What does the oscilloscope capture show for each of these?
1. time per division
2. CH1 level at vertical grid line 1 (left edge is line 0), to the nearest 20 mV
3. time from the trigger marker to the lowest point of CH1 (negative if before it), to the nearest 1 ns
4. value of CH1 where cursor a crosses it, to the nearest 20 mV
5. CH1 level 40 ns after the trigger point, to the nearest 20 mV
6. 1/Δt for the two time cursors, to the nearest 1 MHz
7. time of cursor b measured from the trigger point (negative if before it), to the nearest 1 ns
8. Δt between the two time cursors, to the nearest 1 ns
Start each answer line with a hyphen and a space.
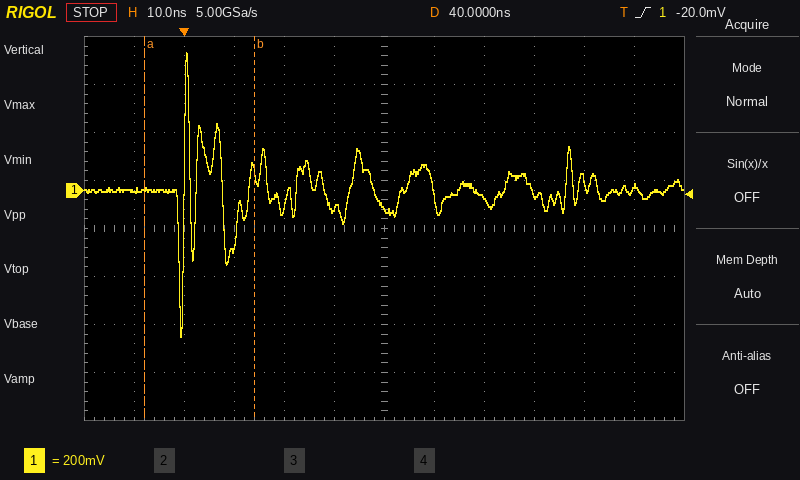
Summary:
- 10 ns
- 0 mV
- -1 ns
- 0 mV
- -80 mV
- 45 MHz
- +14 ns
- 22 ns
